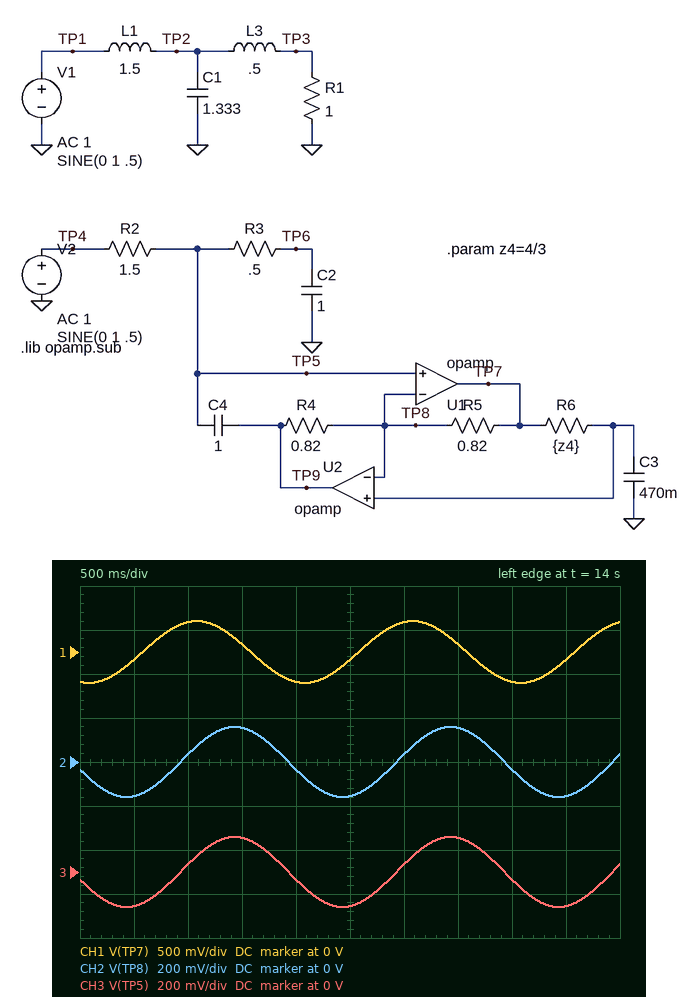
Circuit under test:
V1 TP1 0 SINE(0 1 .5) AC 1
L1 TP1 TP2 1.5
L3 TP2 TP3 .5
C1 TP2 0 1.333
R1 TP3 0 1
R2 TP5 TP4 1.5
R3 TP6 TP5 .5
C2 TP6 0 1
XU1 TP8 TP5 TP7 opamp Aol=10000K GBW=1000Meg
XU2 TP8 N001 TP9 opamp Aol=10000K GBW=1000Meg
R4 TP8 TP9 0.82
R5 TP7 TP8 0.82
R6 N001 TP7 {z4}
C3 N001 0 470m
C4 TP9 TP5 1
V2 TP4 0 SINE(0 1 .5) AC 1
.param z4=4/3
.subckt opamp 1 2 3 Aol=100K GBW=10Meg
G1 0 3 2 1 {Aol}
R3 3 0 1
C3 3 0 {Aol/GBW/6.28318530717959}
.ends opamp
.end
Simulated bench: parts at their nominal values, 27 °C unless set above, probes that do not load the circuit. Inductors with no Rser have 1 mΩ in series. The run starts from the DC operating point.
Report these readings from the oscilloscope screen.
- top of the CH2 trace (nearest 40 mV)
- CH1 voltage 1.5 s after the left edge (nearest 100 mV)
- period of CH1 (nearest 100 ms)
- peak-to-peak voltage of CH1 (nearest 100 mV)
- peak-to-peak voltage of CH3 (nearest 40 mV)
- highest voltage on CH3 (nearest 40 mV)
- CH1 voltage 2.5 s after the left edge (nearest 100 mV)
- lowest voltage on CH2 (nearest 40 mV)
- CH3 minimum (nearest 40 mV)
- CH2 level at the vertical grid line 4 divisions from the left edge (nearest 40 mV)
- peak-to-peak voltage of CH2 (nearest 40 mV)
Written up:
160 mV
100 mV
2.0 s
700 mV
320 mV
160 mV
-100 mV
-160 mV
-160 mV
-40 mV
320 mV
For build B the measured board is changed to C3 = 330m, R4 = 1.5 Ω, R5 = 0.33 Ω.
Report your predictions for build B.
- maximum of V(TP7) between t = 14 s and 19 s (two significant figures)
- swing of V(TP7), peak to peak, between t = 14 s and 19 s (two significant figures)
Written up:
64 mV
130 mV
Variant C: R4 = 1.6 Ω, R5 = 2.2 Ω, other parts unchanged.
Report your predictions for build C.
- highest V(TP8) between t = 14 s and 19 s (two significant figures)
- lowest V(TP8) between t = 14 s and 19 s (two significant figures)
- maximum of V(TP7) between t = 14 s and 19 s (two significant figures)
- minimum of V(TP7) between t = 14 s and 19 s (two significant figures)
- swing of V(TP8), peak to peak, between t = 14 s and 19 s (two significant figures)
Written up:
260 mV
-260 mV
570 mV
-570 mV
520 mV
